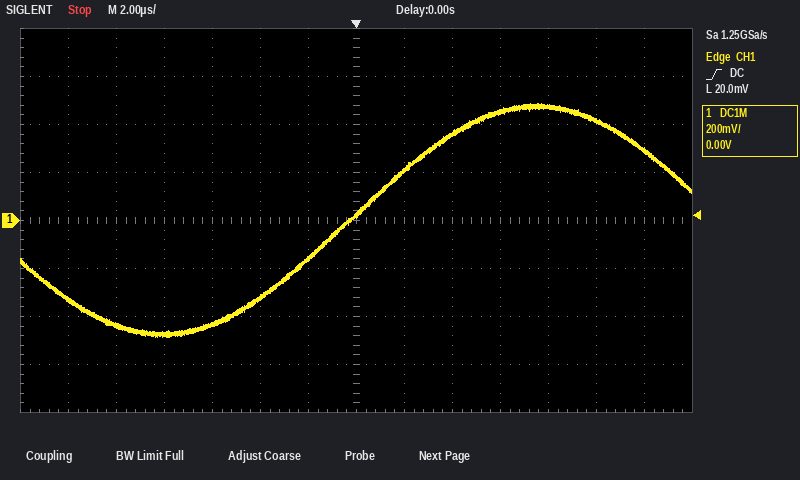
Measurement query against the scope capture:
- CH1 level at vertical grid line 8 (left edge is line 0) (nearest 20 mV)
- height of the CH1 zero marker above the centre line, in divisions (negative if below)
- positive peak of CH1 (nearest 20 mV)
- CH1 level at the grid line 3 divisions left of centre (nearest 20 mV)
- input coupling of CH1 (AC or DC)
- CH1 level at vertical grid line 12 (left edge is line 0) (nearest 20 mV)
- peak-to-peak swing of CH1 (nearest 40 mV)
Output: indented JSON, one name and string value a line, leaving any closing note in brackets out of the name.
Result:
{
  "CH1 level at vertical grid line 8 (left edge is line 0)": "200 mV",
  "height of the CH1 zero marker above the centre line, in divisions": "0.0 div",
  "positive peak of CH1": "480 mV",
  "CH1 level at the grid line 3 divisions left of centre": "-440 mV",
  "input coupling of CH1": "DC",
  "CH1 level at vertical grid line 12 (left edge is line 0)": "420 mV",
  "peak-to-peak swing of CH1": "960 mV"
}
